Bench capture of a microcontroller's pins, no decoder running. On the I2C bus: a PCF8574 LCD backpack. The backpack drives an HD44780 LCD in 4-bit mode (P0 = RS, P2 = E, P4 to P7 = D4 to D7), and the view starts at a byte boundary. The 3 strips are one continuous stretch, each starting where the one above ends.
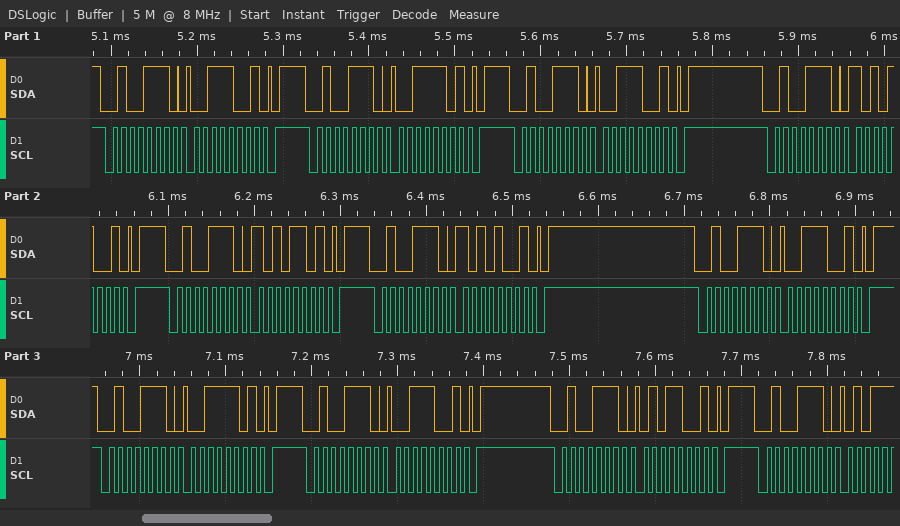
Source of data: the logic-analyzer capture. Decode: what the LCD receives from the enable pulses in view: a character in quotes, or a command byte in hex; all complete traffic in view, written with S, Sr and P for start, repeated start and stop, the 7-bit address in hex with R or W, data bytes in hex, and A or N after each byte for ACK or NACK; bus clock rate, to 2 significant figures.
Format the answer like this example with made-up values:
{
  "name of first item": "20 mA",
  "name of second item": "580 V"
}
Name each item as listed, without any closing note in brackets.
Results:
{
  "what the LCD receives from the enable pulses in view: a character in quotes, or a command byte in hex": "':'",
  "all complete traffic in view, written with S, Sr and P for start, repeated start and stop, the 7-bit address in hex with R or W, data bytes in hex, and A or N after each byte for ACK or NACK": "S 27W A 39 A P S 27W A 3D A P S 27W A 39 A P S 27W A A9 A P S 27W A AD A P S 27W A A9 A P S 27W A 39 A P S 27W A 3D A P S 27W A 39 A P S 27W A 59 A P S 27W A",
  "bus clock rate, to 2 significant figures": "100 kHz"
}
